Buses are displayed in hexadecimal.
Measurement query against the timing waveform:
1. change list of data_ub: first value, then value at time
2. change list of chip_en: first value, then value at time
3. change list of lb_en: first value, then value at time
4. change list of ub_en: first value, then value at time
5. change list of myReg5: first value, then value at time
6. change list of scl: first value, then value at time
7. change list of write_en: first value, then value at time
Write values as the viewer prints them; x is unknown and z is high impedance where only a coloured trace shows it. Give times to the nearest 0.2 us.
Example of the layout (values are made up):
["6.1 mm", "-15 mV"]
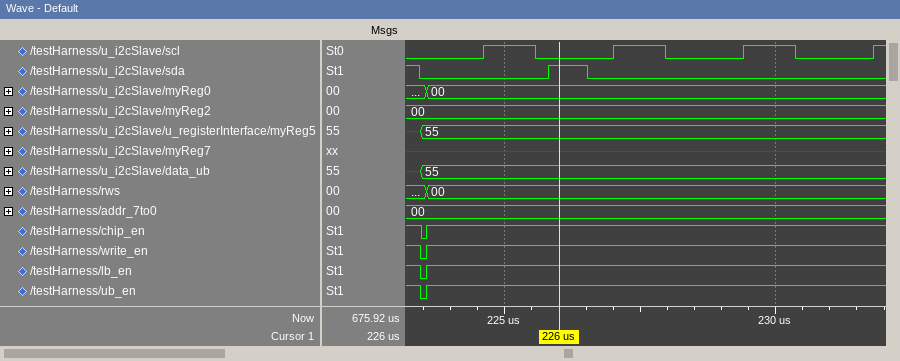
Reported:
["x, 55 at 223.4 us", "1, 0 at 223.4 us, 1 at 223.6 us", "1, 0 at 223.4 us, 1 at 223.6 us", "1, 0 at 223.4 us, 1 at 223.6 us", "x, 55 at 223.4 us", "0, 1 at 224.6 us, 0 at 225.6 us, 1 at 227 us, 0 at 228 us, 1 at 229.4 us, 0 at 230.4 us, 1 at 231.8 us", "1, 0 at 223.4 us, 1 at 223.6 us"]
